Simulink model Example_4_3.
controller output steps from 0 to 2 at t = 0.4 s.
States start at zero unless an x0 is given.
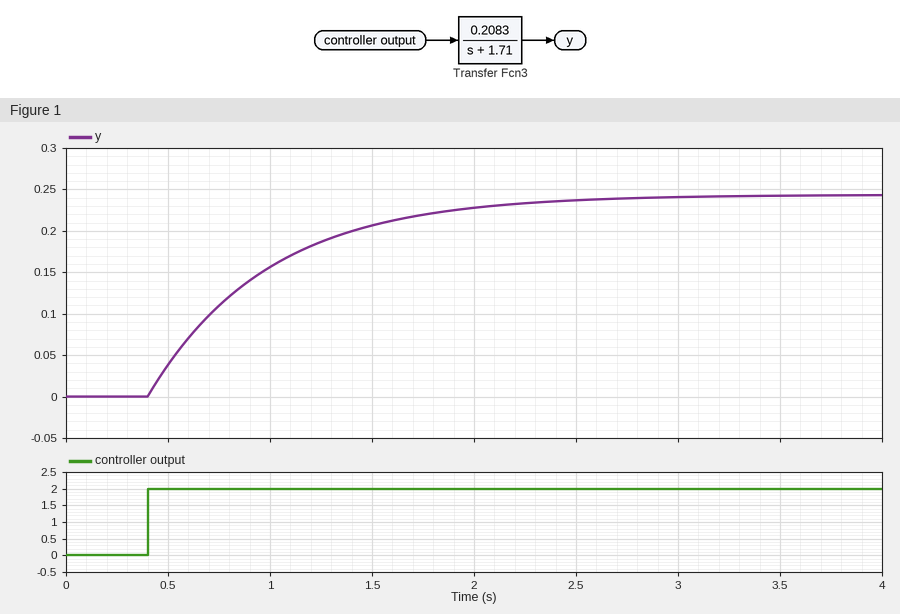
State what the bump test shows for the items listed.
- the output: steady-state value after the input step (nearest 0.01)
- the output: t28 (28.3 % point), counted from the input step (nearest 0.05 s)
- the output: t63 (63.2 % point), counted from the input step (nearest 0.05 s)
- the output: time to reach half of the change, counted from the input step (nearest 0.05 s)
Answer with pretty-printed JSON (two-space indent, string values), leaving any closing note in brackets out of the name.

{
  "the output: steady-state value after the input step": "0.24",
  "the output: t28 (28.3 % point), counted from the input step": "0.20 s",
  "the output: t63 (63.2 % point), counted from the input step": "0.60 s",
  "the output: time to reach half of the change, counted from the input step": "0.40 s"
}
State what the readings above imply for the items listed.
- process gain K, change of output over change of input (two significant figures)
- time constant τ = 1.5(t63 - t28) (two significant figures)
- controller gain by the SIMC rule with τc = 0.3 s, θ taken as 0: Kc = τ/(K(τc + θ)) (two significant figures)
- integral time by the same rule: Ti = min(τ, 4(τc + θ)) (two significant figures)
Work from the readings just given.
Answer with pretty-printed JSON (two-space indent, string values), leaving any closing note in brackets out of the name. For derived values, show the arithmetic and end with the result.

{
  "process gain K, change of output over change of input": "(0.24 - 0) / 2 = 0.12",
  "time constant τ = 1.5(t63 - t28)": "1.5 × (0.6 - 0.2) = 0.60 s",
  "controller gain by the SIMC rule with τc = 0.3 s, θ taken as 0: Kc = τ/(K(τc + θ))": "0.6 / (0.12 × (0.3 + 0)) = 17",
  "integral time by the same rule: Ti = min(τ, 4(τc + θ))": "min(0.6, 4 × (0.3 + 0)) = 0.60 s"
}
